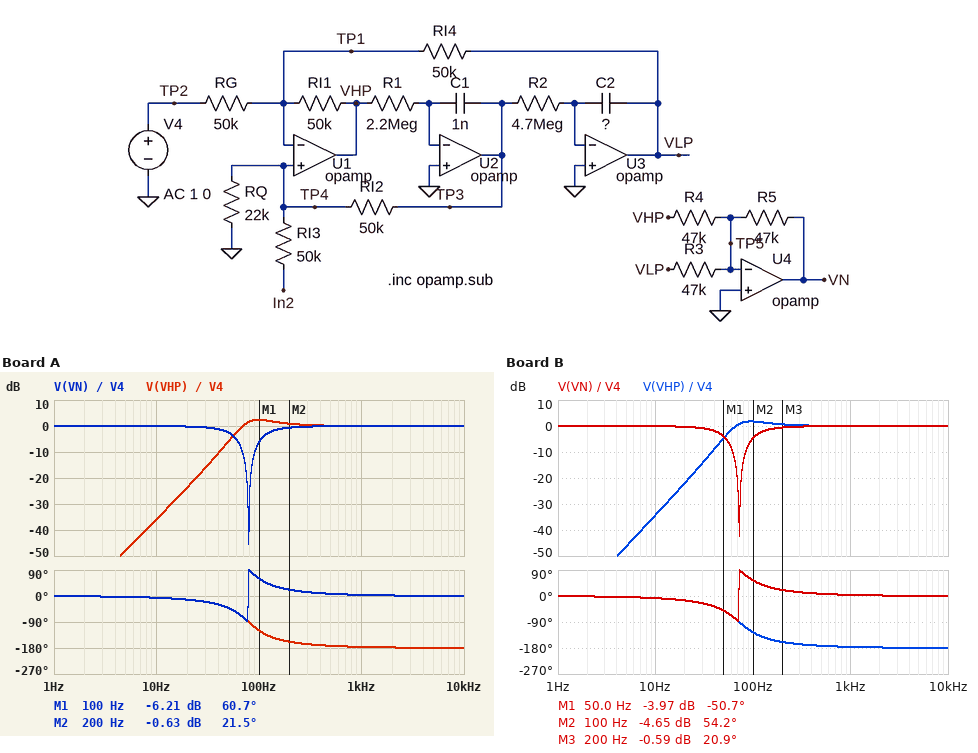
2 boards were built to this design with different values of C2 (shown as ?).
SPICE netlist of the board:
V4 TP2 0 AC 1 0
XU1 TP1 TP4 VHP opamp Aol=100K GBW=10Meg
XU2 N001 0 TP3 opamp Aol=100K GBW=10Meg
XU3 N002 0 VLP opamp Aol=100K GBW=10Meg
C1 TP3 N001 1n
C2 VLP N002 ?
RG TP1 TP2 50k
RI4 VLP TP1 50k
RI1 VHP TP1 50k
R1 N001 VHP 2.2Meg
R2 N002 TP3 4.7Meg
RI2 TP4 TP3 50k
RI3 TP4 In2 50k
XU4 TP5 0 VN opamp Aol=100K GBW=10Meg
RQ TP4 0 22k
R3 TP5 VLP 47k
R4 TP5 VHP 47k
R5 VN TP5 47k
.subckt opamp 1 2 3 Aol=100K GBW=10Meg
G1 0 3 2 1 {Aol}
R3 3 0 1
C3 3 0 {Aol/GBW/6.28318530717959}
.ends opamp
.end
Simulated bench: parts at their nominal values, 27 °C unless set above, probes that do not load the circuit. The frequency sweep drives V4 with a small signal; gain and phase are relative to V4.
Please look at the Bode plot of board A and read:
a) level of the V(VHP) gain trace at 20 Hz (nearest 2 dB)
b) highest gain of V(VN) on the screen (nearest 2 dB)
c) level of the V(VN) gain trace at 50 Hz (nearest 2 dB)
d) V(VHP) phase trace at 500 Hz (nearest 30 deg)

-24 dB
0 dB
-2 dB
-180 deg
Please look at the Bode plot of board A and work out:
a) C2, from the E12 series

390 pF
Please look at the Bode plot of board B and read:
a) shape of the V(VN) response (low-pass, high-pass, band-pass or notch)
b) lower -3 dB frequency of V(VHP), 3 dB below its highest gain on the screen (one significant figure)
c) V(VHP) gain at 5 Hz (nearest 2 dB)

notch
60 Hz
-46 dB
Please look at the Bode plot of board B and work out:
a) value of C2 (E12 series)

470 pF
